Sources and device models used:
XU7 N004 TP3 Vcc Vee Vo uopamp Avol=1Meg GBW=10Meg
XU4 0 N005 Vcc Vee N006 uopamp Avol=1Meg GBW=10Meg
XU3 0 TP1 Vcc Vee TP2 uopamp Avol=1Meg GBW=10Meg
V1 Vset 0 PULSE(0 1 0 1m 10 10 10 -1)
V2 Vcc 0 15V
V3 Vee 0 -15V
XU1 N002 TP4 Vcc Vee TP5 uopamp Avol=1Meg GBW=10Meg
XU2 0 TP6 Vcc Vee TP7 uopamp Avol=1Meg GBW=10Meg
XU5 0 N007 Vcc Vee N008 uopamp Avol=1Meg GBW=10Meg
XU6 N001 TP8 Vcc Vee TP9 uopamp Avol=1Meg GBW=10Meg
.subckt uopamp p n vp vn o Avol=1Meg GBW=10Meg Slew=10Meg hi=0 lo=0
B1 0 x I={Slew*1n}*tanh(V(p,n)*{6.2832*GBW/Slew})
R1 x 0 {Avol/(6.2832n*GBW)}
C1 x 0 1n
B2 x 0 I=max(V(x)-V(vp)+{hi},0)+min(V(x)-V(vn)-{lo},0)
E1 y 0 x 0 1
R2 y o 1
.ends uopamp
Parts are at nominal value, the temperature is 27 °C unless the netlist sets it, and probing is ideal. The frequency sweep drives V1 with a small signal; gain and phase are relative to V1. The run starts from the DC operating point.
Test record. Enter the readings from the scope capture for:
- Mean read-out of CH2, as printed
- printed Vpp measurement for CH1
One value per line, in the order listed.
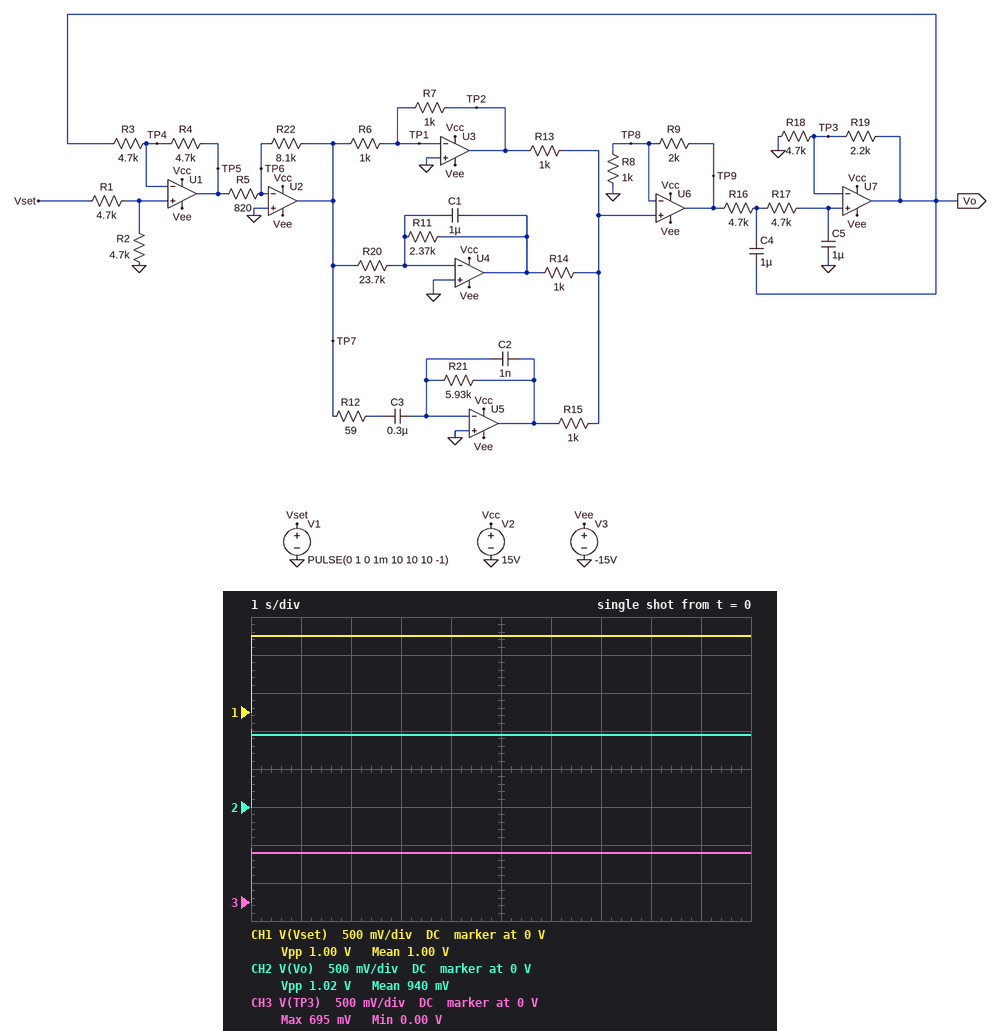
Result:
940 mV
1.00 V
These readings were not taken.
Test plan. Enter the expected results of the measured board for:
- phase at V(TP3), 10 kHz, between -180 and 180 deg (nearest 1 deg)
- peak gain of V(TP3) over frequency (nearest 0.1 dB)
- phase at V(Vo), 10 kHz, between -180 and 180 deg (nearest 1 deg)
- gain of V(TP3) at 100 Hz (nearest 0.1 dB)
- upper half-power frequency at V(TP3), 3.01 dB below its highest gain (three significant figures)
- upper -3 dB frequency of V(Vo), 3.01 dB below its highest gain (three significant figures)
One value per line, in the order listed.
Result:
-164 deg
-3.1 dB
-164 deg
-3.2 dB
229 Hz
229 Hz
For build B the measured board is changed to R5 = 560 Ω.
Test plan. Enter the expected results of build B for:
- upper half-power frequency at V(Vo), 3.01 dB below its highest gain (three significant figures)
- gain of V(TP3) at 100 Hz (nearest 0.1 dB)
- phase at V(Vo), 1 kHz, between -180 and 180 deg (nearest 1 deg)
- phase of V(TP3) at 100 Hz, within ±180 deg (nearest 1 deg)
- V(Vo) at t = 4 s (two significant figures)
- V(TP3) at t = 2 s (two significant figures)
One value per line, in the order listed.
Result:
316 Hz
-3.1 dB
-85 deg
-16 deg
960 mV
650 mV
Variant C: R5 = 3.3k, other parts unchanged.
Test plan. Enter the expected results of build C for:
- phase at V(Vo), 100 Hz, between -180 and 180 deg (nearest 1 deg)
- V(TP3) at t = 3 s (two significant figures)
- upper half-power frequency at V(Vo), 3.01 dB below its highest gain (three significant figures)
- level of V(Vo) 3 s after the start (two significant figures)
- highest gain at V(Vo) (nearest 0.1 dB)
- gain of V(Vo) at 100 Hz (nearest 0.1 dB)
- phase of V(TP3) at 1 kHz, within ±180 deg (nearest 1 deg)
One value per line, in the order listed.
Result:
-70 deg
540 mV
94.8 Hz
800 mV
-1.2 dB
-4.7 dB
-98 deg
